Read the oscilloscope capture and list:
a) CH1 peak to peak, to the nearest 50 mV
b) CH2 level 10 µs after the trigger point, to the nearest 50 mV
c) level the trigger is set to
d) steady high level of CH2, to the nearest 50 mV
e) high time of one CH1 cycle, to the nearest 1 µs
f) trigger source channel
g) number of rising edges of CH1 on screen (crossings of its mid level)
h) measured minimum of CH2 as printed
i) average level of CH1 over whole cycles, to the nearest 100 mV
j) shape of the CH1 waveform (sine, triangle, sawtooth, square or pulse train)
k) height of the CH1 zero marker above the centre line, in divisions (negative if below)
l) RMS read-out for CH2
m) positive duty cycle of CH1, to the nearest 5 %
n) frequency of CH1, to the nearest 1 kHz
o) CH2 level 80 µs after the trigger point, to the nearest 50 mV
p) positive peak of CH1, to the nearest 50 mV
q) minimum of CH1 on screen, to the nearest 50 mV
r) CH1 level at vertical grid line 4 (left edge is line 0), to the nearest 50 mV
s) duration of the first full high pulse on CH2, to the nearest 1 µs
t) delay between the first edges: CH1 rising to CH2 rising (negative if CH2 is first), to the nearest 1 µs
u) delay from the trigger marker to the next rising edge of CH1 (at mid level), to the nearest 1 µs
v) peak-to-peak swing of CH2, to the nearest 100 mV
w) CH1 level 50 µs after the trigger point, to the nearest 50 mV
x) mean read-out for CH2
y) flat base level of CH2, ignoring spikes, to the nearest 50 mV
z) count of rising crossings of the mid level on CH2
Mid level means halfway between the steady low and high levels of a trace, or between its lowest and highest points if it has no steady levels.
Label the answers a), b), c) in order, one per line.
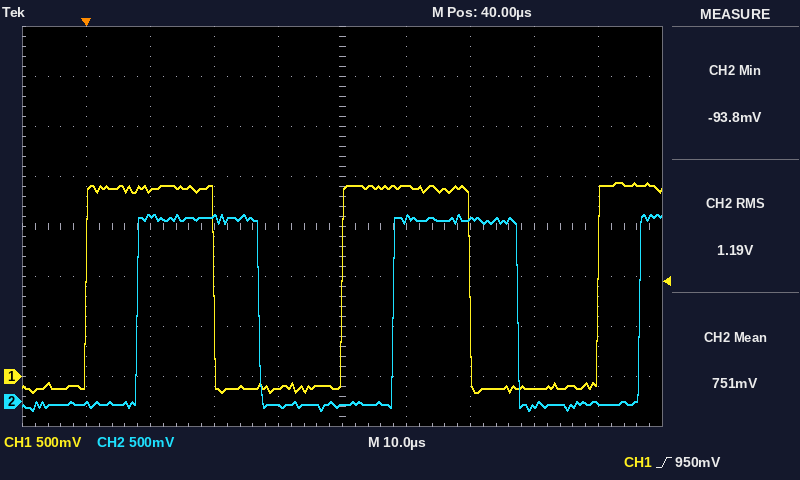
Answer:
a) 2.10 V
b) 1.85 V
c) 950 mV
d) 1.85 V
e) 20 µs
f) CH1
g) 3
h) -93.8 mV
i) 900 mV
j) square
k) -3.0 div
l) 1.19 V
m) 50 %
n) 25 kHz
o) 0 mV
p) 1.95 V
q) -150 mV
r) -100 mV
s) 19 µs
t) +8 µs
u) 40 µs
v) 2.00 V
w) 1.90 V
x) 751 mV
y) -50 mV
z) 3
